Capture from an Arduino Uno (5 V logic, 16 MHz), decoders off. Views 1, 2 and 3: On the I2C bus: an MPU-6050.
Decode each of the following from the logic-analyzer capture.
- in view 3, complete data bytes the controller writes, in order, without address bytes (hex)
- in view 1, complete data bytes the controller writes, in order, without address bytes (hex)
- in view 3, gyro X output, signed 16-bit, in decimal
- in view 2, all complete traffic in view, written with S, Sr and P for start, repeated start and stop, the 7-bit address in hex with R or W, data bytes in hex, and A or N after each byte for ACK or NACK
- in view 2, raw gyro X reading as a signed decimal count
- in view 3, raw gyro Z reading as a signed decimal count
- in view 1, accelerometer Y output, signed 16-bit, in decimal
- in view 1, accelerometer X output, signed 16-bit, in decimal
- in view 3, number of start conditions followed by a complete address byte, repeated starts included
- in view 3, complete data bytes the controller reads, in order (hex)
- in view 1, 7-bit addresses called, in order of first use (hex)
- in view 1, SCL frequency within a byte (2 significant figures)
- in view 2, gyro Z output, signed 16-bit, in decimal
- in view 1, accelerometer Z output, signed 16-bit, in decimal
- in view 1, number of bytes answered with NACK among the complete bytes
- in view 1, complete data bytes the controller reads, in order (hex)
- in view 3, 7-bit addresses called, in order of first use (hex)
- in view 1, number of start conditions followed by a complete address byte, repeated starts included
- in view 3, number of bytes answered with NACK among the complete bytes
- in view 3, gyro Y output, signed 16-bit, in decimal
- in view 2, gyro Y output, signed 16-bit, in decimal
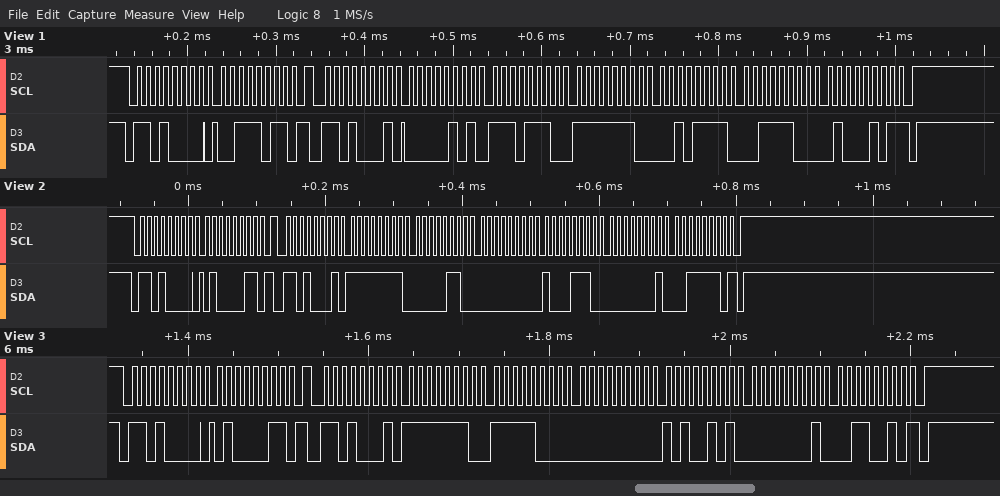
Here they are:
43
3B
-264
S 68W A 43 A Sr 68R A FF A 06 A 00 A 8E A 01 A 3E N P
-250
306
-465
1518
2
FE F8 00 A5 01 32
0x68
100 kHz
318
15429
1
05 EE FE 2F 3C 45
0x68
2
1
165
142
